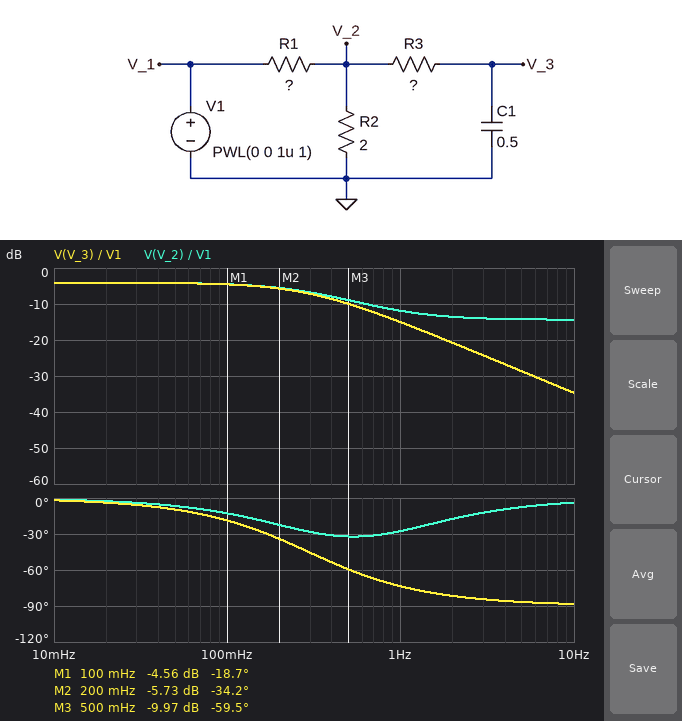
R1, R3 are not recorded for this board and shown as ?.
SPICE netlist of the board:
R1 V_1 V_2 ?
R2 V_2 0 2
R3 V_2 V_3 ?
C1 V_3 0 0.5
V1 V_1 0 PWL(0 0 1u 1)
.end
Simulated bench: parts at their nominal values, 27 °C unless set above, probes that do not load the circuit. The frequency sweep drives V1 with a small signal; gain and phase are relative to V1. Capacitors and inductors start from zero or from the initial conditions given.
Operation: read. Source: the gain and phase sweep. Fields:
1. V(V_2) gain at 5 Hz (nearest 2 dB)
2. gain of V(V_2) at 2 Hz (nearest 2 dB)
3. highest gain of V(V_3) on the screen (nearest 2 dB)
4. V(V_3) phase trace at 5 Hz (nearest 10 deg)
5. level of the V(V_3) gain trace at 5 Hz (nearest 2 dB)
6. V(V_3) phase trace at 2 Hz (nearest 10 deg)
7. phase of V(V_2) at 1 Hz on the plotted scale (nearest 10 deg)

-14 dB
-14 dB
-4 dB
-90 deg
-28 dB
-80 deg
-30 deg
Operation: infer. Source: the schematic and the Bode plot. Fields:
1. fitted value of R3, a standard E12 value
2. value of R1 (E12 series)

0.33 Ω
1.2 Ω
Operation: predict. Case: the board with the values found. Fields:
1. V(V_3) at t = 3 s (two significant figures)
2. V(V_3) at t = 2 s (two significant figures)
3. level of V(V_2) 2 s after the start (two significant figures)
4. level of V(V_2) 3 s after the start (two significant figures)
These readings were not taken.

620 mV
610 mV
610 mV
620 mV
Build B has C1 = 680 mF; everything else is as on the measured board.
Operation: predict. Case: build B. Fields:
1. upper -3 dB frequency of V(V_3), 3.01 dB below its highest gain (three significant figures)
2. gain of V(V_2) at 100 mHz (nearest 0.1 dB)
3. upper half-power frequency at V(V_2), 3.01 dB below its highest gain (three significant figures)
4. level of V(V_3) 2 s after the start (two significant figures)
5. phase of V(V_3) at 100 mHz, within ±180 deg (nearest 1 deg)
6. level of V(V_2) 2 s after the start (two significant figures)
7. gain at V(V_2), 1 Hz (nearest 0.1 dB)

217 mHz
-4.8 dB
240 mHz
580 mV
-25 deg
600 mV
-12.8 dB
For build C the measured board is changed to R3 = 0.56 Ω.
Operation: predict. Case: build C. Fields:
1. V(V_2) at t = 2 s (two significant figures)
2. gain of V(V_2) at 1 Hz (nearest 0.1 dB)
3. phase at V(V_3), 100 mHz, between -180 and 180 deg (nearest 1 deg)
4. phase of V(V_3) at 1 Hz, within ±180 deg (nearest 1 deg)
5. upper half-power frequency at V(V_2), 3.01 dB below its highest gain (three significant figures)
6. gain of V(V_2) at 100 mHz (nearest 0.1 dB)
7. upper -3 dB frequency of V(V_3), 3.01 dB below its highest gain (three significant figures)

610 mV
-10.5 dB
-22 deg
-76 deg
305 mHz
-4.6 dB
243 mHz
